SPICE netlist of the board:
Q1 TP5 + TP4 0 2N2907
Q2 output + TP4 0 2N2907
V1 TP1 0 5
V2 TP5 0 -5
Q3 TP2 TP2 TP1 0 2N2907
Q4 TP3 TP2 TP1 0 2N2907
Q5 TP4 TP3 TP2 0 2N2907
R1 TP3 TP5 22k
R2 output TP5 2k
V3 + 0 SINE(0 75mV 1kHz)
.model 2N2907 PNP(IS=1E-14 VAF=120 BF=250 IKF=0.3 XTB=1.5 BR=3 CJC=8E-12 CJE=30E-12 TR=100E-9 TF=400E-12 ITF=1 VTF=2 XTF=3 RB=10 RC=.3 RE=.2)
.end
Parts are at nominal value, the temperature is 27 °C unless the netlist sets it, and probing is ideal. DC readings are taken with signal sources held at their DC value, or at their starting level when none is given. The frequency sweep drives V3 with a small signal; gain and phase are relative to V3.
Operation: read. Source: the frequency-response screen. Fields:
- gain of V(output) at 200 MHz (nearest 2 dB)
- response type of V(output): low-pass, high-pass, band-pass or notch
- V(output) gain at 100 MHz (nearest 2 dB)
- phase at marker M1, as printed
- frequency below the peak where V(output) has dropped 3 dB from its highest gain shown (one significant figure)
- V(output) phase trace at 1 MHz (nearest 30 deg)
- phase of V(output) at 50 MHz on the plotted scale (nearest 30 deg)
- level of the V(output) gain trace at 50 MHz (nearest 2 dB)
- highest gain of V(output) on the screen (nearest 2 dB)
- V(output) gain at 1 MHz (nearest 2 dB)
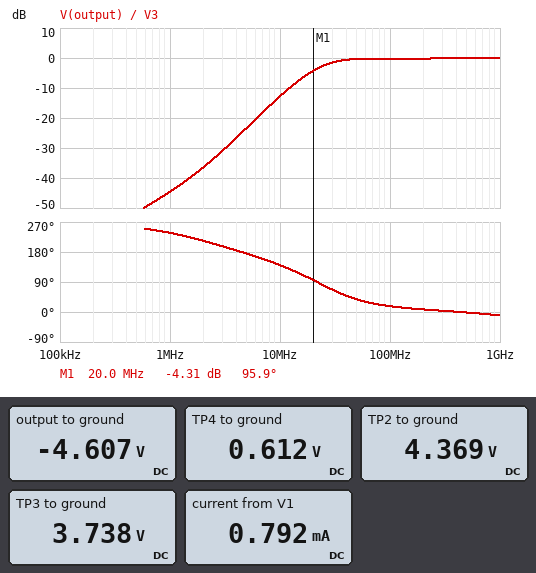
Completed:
0 dB
high-pass
0 dB
95.9 deg
20 MHz
240 deg
30 deg
0 dB
0 dB
-44 dB
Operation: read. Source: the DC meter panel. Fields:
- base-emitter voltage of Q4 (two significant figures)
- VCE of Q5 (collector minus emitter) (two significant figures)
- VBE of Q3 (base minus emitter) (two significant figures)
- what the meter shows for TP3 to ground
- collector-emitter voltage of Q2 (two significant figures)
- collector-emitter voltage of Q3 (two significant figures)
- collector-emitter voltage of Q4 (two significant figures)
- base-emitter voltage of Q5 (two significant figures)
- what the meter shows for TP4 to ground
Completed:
-630 mV
-3.8 V
-630 mV
3.738 V
-5.2 V
-630 mV
-1.3 V
-630 mV
0.612 V
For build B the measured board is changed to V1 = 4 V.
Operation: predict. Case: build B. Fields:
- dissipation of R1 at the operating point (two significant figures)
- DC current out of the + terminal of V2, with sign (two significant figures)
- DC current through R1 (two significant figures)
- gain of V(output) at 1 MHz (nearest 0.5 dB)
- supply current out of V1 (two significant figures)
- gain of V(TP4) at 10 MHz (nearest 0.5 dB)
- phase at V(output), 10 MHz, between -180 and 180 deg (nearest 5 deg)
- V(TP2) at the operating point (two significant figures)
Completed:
2.7 mW
-700 µA
350 µA
-38.5 dB
700 µA
0 dB
145 deg
3.4 V
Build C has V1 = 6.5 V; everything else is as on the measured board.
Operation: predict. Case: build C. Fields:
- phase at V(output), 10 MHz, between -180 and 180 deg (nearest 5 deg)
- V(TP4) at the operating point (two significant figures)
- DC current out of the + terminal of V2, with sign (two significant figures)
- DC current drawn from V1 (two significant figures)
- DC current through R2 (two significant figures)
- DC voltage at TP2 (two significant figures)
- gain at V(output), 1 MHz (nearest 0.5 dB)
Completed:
130 deg
620 mV
-930 µA
930 µA
230 µA
5.9 V
-52.5 dB
